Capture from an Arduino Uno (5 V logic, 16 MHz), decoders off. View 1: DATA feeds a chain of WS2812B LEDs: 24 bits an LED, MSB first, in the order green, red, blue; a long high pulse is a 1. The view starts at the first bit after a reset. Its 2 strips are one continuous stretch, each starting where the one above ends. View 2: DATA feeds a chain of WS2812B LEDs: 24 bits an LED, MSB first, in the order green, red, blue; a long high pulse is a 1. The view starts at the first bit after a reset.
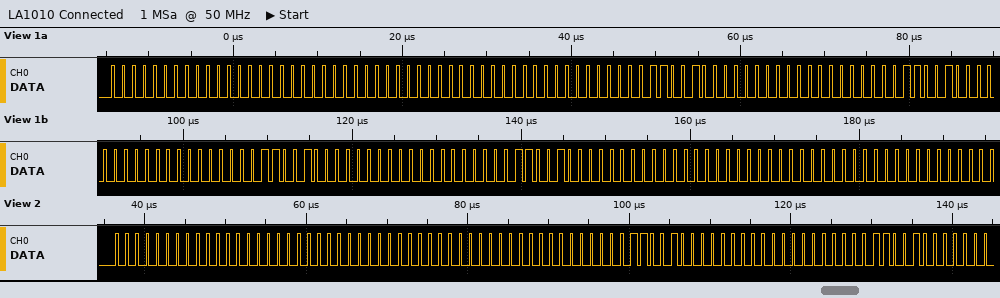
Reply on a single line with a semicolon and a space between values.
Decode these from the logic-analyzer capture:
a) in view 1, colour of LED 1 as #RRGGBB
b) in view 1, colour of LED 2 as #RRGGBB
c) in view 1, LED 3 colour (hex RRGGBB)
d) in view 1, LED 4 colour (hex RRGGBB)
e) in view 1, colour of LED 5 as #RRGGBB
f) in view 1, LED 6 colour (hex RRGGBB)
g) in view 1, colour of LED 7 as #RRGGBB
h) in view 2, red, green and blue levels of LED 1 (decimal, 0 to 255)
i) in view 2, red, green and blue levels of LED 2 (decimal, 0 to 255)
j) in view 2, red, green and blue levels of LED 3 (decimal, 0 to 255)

#000000; #000000; #001900; #001900; #001900; #001900; #000000; 0, 0, 0; 0, 0, 0; 0, 25, 0
